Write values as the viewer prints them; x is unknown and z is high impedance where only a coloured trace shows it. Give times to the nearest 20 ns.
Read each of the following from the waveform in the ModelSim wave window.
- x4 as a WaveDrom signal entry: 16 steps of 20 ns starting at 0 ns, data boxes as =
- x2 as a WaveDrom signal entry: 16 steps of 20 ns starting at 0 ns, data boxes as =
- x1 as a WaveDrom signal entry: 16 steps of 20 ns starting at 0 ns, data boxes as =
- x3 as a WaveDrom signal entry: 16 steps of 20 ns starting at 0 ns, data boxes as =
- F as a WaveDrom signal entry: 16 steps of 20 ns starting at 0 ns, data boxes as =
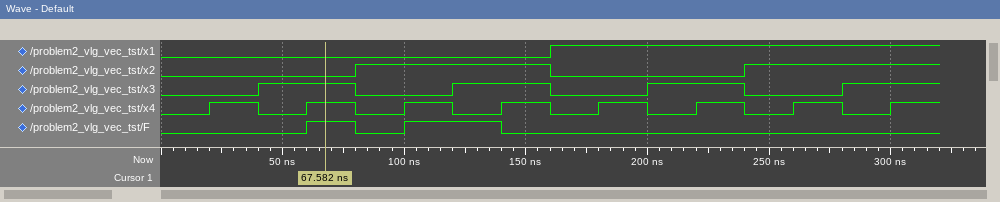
{name: 'x4', wave: '0101010101010101'}
{name: 'x2', wave: '0...1...0...1...'}
{name: 'x1', wave: '0.......1.......'}
{name: 'x3', wave: '0.1.0.1.0.1.0.1.'}
{name: 'F', wave: '0..101.0........'}
